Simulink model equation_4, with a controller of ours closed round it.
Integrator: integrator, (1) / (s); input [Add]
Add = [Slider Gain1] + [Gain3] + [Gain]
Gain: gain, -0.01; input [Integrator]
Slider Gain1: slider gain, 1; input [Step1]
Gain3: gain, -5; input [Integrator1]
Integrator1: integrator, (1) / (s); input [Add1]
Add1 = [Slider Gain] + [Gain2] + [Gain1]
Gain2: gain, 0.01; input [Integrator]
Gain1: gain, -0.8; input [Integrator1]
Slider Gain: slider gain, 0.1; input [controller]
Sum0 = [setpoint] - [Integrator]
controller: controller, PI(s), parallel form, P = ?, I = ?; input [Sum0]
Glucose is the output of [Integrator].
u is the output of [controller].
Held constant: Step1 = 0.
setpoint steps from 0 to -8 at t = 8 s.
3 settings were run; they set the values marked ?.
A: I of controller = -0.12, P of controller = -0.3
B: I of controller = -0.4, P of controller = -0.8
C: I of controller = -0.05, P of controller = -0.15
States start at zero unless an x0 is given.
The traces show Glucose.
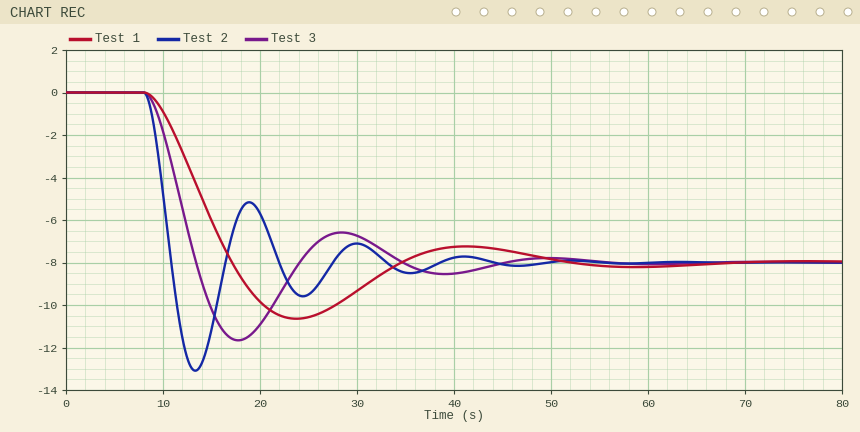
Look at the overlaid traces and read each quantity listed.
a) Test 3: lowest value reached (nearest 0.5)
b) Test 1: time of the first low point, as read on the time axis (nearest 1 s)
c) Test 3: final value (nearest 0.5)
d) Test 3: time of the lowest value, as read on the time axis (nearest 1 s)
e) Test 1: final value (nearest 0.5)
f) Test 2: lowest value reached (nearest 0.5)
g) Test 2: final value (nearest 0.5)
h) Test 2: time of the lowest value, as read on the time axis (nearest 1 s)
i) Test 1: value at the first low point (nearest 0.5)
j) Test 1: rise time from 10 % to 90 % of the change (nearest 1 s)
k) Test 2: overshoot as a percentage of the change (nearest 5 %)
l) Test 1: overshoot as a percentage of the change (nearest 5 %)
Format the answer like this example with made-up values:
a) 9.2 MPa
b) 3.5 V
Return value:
a) -11.5
b) 24 s
c) -8.0
d) 18 s
e) -8.0
f) -13.0
g) -8.0
h) 13 s
i) -10.5
j) 6 s
k) 65 %
l) 35 %
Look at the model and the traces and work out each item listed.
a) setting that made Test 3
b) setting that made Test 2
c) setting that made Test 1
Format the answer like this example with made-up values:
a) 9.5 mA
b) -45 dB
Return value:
a) A
b) B
c) C
